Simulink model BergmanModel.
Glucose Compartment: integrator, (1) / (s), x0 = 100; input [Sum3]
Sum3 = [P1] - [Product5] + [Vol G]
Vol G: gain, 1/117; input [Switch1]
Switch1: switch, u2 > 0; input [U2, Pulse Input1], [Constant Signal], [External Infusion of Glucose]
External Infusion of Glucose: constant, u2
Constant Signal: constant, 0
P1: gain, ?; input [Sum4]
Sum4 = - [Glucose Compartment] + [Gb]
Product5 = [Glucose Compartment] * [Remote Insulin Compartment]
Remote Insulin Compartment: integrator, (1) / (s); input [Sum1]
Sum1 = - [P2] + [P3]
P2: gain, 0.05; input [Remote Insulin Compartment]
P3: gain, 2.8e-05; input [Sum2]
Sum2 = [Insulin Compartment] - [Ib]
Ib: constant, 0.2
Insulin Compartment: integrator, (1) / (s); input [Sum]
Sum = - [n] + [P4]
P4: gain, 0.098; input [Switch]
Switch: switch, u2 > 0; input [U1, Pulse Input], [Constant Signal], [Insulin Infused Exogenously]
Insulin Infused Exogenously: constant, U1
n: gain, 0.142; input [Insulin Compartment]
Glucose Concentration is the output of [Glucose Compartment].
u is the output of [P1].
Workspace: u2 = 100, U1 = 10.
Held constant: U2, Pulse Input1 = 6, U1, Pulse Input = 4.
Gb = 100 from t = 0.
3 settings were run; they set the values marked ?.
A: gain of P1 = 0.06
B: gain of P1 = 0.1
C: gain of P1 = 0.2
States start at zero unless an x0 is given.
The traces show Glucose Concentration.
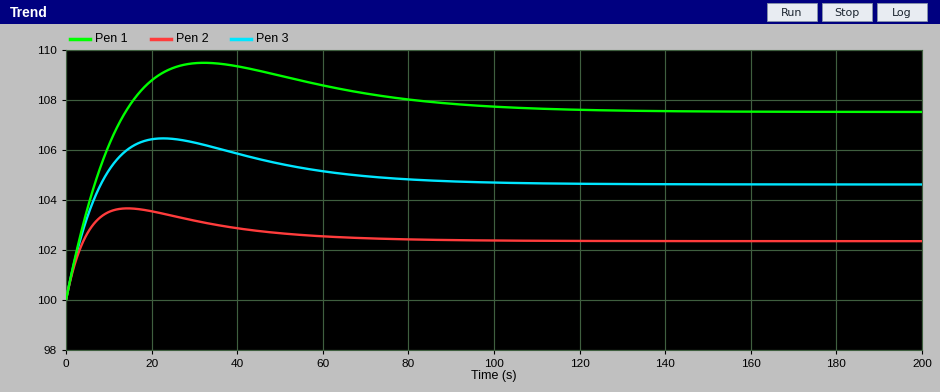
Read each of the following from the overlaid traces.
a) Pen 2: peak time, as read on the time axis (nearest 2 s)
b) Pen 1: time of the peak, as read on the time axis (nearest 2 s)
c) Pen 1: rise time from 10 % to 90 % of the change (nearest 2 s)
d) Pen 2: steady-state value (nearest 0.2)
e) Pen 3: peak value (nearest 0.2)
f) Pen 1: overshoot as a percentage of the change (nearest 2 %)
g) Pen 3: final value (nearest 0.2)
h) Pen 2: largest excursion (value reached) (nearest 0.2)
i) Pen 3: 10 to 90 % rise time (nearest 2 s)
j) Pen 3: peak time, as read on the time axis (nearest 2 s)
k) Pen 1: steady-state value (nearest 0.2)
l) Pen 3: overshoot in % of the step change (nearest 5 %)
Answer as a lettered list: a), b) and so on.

a) 14 s
b) 32 s
c) 10 s
d) 102.4
e) 106.4
f) 26 %
g) 104.6
h) 103.6
i) 6 s
j) 22 s
k) 107.6
l) 40 %
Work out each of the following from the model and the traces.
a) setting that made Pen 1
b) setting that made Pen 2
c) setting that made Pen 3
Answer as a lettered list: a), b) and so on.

a) A
b) C
c) B
